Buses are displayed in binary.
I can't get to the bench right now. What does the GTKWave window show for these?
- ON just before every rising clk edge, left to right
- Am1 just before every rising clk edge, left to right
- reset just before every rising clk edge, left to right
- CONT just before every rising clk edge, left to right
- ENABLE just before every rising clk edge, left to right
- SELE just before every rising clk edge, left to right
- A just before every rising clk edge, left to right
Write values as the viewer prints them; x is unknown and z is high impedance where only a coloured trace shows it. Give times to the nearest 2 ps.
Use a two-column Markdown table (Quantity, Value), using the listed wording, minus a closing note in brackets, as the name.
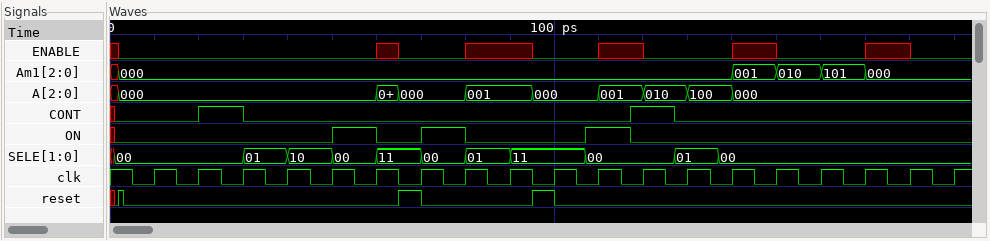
| Quantity | Value |
|---|---|
| ON just before every rising clk edge, left to right | 0 0 0 0 0 1 0 1 0 0 1 0 0 0 0 0 0 0 0 |
| Am1 just before every rising clk edge, left to right | 000, 000, 000, 000, 000, 000, 000, 000, 000, 000, 000, 000, 000, 000, 001, 010, 101, 000, 000 |
| reset just before every rising clk edge, left to right | 0 0 0 0 0 0 1 0 0 1 0 0 0 0 0 0 0 0 0 |
| CONT just before every rising clk edge, left to right | 0 0 1 0 0 0 0 0 0 0 0 1 0 0 0 0 0 0 0 |
| ENABLE just before every rising clk edge, left to right | 0 0 0 0 0 0 0 0 x 0 0 x 0 0 x 0 0 x 0 |
| SELE just before every rising clk edge, left to right | 00, 00, 00, 01, 10, 00, 11, 00, 01, 11, 00, 00, 01, 00, 00, 00, 00, 00, 00 |
| A just before every rising clk edge, left to right | 000, 000, 000, 000, 000, 000, 000, 000, 001, 000, 000, 001, 010, 100, 000, 000, 000, 000, 000 |
